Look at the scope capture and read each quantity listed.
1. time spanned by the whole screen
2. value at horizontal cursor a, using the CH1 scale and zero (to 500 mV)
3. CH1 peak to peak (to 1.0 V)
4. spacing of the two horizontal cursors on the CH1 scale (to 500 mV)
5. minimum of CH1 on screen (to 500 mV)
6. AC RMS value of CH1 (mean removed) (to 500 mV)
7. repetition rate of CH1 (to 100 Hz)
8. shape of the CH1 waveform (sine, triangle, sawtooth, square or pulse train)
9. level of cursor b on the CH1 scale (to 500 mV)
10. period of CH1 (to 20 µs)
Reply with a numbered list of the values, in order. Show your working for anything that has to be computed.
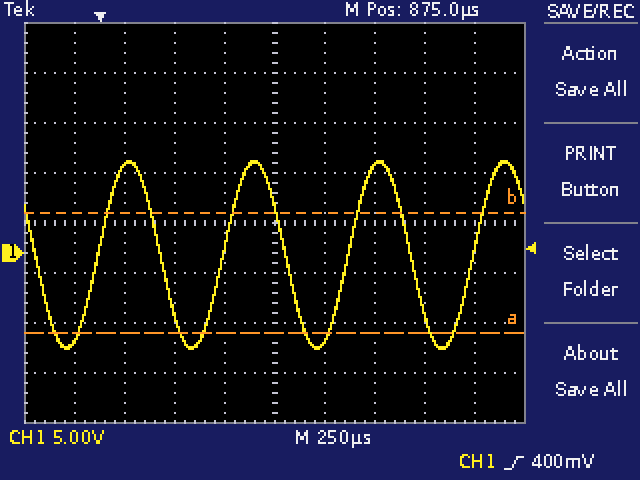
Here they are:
1. 2.5 ms
2. -8.0 V
3. 19.0 V
4. 12.0 V
5. -9.5 V
6. 19.0 V / (2√2) ≈ 6.72 V, so 6.5 V to the nearest 500 mV
7. 1 / 620 µs ≈ 1.6 kHz
8. sine
9. 4.0 V
10. 620 µs
